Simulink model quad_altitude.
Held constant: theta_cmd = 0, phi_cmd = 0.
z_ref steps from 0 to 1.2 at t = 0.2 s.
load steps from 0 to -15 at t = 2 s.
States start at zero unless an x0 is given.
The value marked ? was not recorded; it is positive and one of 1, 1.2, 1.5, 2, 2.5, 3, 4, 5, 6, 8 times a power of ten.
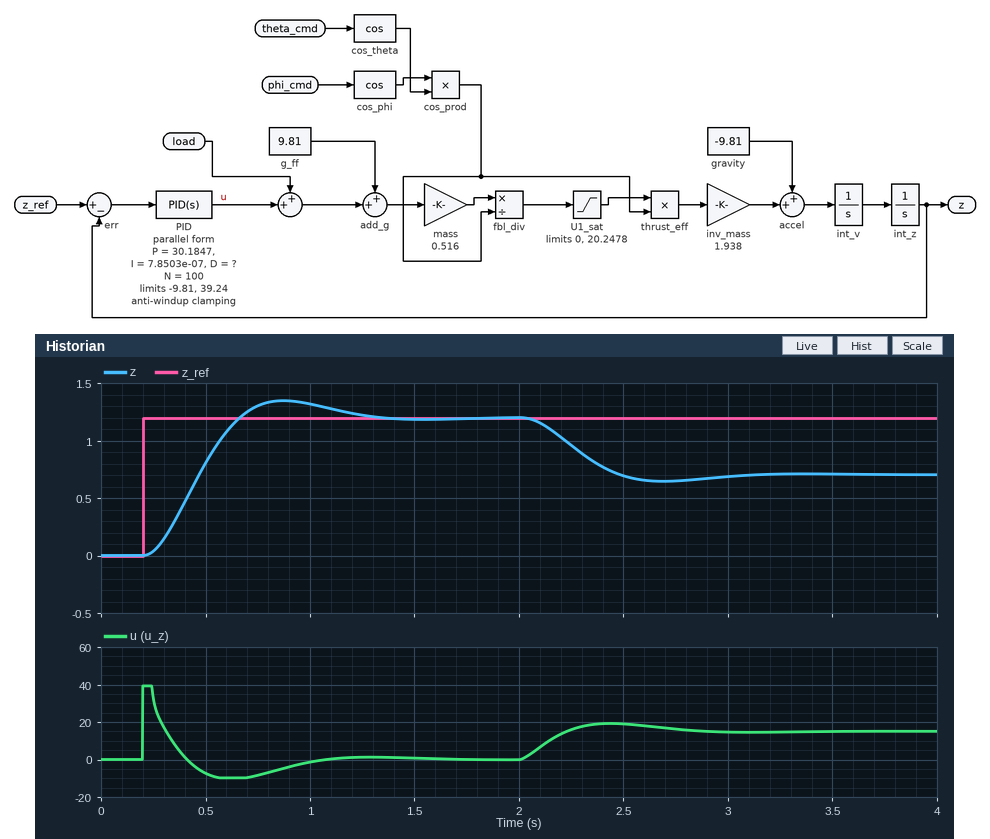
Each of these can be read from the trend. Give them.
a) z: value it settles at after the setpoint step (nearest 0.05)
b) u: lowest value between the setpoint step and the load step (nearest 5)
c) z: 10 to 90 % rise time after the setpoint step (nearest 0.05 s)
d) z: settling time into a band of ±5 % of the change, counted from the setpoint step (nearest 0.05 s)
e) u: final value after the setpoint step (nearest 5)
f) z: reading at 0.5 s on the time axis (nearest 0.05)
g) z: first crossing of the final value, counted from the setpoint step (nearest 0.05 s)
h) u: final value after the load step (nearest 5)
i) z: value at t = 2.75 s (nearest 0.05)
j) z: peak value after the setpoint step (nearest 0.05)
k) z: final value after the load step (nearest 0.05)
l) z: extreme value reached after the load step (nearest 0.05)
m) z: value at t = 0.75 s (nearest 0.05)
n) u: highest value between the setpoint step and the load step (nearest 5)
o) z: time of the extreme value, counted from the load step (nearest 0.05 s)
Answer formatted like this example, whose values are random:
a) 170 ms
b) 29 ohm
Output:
a) 1.20
b) -10
c) 0.30 s
d) 0.95 s
e) 0
f) 0.80
g) 0.45 s
h) 15
i) 0.65
j) 1.35
k) 0.70
l) 0.65
m) 1.30
n) 40
o) 0.70 s
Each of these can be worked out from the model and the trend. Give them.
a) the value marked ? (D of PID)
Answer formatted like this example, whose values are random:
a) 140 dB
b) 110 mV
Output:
a) 6
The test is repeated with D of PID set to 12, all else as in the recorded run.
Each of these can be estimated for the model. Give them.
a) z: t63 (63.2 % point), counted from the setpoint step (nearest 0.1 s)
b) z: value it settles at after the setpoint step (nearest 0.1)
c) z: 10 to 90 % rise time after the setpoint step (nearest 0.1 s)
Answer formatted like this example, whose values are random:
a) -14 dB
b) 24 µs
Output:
a) 0.4 s
b) 1.2
c) 0.7 s
